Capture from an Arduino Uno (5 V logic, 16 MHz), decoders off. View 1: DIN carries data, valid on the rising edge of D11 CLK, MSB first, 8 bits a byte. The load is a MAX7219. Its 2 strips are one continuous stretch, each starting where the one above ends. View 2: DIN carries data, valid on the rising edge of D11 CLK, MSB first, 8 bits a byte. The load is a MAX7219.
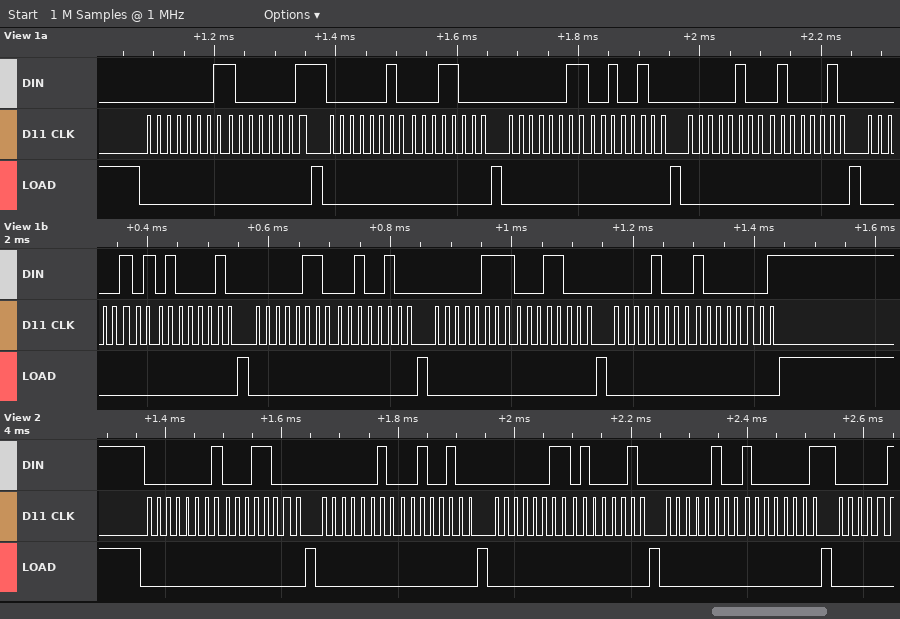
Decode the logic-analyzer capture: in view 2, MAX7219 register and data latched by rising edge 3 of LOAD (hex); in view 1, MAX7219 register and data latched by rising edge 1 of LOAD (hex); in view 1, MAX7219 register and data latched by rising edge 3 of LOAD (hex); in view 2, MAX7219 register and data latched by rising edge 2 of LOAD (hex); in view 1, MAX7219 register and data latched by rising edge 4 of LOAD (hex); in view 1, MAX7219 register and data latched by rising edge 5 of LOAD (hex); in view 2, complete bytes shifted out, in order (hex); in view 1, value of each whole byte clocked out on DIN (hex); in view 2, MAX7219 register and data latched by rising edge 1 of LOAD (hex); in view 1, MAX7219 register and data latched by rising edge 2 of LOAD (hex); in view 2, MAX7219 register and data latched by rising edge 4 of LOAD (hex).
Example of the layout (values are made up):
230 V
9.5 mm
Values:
register 0x3, data 0x42
register 0x1, data 0x81
register 0x3, data 0x24
register 0x2, data 0x24
register 0x4, data 0x42
register 0x5, data 0x42
0x01 0x18 0x02 0x24 0x03 0x42 0x04 0x81
01 81 02 18 03 24 04 42 05 42 06 24 07 18 08 81
register 0x1, data 0x18
register 0x2, data 0x18
register 0x4, data 0x81
